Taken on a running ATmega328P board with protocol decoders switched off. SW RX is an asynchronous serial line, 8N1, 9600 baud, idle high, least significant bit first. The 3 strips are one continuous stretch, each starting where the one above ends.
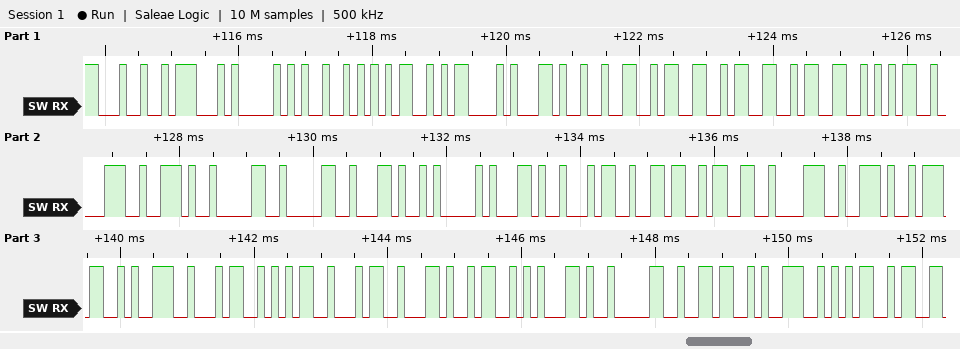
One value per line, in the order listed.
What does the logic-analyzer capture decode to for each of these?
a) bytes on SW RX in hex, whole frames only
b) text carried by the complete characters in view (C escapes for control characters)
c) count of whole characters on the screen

24 47 50 52 4D 43 2C 32 33 33 33 35 38 2E 30 30 2C 41 2C 34 36 33 38 2E 37 39 34 35 34 2C 53 2C 30 36 39 35
"$GPRMC,233358.00,A,4638.79454,S,0695"
36
